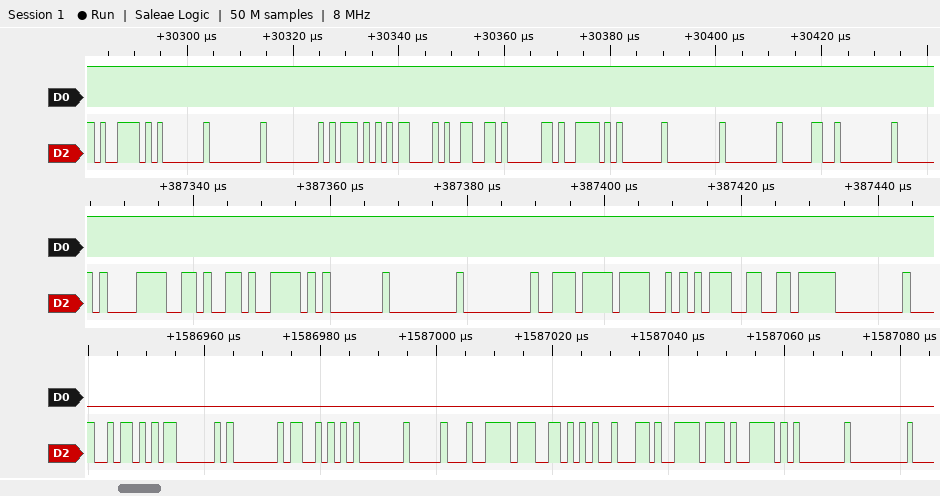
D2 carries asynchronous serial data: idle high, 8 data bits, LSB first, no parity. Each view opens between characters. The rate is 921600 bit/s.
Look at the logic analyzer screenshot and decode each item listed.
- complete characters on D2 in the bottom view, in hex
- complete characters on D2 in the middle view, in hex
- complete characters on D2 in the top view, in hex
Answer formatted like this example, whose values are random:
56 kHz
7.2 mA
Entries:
5A, 03, 01, 53, 01, 10, DE, 56, 62, DE, 79, 01, 00
E1, 96, 79, 01, 00, 00, EE, 4F, 9D, F6, 00
79, 01, 00, 00, 5D, 0D, 99, 81, 79, 01, 00, 00, 30, 00
